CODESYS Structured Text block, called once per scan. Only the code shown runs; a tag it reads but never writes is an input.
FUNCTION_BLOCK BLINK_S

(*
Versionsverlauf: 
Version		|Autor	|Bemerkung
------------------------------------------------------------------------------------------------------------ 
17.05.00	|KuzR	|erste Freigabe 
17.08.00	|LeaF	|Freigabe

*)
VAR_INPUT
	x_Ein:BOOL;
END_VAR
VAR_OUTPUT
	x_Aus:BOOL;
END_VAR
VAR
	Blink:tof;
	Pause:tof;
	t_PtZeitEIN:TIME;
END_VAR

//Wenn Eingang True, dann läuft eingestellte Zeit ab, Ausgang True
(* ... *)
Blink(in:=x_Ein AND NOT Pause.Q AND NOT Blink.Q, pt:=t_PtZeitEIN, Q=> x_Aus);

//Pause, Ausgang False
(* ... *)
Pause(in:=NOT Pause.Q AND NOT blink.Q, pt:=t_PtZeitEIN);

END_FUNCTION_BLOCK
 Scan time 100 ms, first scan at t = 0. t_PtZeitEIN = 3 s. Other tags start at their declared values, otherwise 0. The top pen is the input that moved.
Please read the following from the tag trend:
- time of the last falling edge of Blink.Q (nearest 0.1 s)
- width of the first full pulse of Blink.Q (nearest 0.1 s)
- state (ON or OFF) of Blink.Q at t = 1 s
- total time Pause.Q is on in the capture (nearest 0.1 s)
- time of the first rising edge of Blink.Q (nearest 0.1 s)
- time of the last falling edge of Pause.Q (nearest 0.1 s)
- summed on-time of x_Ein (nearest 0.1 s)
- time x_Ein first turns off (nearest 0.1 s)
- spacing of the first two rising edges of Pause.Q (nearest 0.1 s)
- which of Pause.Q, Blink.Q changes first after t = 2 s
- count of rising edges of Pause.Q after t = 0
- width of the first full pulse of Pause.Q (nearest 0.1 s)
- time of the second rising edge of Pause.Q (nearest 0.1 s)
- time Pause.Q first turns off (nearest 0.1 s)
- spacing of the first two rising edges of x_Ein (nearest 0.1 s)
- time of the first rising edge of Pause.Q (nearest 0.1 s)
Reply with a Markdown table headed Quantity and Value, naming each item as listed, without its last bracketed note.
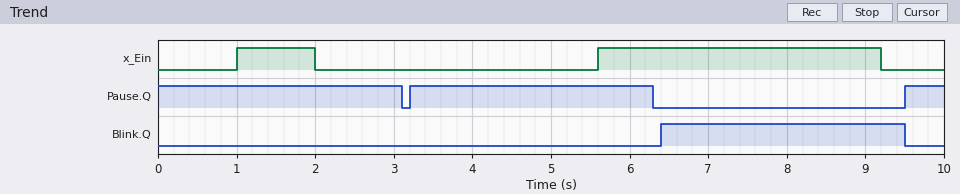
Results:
| Quantity | Value |
|---|---|
| time of the last falling edge of Blink.Q | 9.5 s |
| width of the first full pulse of Blink.Q | 3.1 s |
| state (ON or OFF) of Blink.Q at t = 1 s | OFF |
| total time Pause.Q is on in the capture | 6.7 s |
| time of the first rising edge of Blink.Q | 6.4 s |
| time of the last falling edge of Pause.Q | 6.3 s |
| summed on-time of x_Ein | 4.6 s |
| time x_Ein first turns off | 2.0 s |
| spacing of the first two rising edges of Pause.Q | 6.3 s |
| which of Pause.Q, Blink.Q changes first after t = 2 s | Pause.Q |
| count of rising edges of Pause.Q after t = 0 | 2 |
| width of the first full pulse of Pause.Q | 3.1 s |
| time of the second rising edge of Pause.Q | 9.5 s |
| time Pause.Q first turns off | 3.1 s |
| spacing of the first two rising edges of x_Ein | 4.6 s |
| time of the first rising edge of Pause.Q | 3.2 s |
